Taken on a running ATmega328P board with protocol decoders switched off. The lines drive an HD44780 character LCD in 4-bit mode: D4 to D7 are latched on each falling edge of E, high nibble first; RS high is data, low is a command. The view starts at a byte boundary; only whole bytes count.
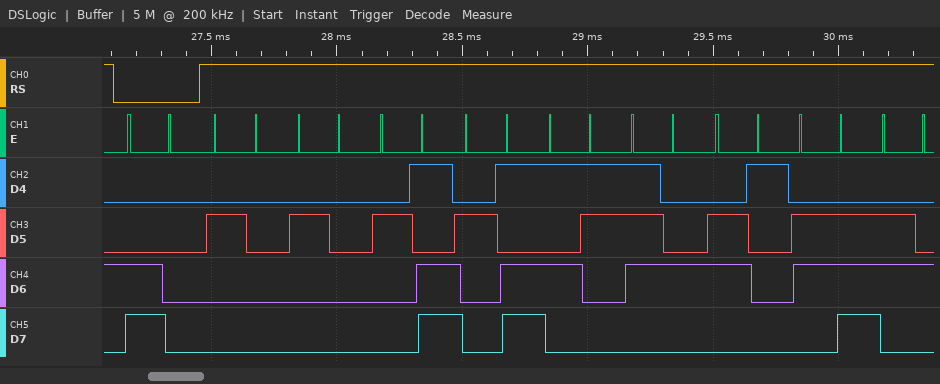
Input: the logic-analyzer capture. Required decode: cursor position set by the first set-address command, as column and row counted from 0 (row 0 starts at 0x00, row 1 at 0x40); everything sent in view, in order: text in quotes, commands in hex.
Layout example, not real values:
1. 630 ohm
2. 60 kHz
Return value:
1. column 0, row 1
2. 0xC0 "  --Stand"
